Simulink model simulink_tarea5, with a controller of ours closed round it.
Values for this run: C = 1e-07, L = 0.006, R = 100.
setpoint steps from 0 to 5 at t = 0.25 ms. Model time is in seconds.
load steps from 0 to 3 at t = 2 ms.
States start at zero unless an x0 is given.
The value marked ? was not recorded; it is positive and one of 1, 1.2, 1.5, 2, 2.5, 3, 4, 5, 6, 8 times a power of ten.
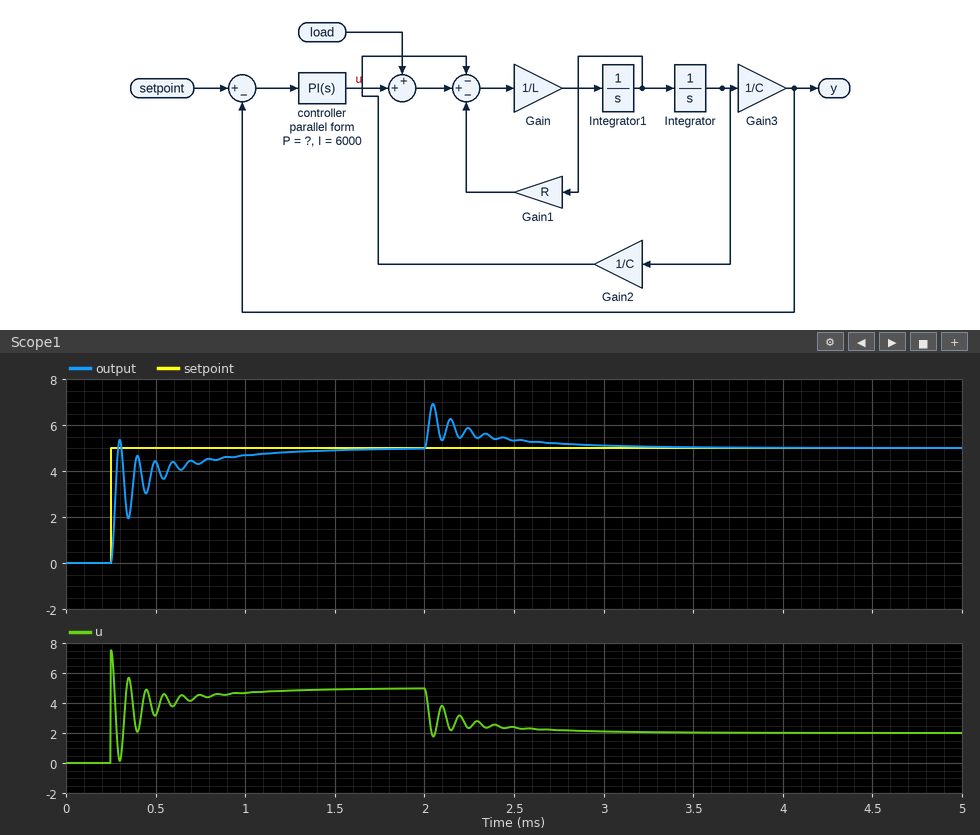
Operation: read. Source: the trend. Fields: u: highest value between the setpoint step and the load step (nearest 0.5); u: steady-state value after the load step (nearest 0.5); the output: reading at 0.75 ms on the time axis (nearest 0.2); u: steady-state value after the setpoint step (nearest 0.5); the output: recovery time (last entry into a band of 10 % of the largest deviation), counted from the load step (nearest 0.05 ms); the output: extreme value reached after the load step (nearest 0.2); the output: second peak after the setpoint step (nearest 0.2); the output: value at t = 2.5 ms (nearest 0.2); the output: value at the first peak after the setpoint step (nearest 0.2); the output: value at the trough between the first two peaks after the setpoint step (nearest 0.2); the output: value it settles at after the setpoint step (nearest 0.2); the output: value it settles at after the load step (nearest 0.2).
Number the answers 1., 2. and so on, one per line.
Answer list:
1. 7.5
2. 2.0
3. 4.4
4. 5.0
5. 0.75 ms
6. 7.0
7. 4.6
8. 5.4
9. 5.4
10. 2.0
11. 5.0
12. 5.0
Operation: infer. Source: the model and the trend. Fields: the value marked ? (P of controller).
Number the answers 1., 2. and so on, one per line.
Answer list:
1. 1.5
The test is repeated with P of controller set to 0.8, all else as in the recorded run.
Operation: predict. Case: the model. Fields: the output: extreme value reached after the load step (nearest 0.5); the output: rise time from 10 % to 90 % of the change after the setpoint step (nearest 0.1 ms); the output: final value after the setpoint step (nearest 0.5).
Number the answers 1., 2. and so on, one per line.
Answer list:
1. 7.5
2. 0.5 ms
3. 5.0
